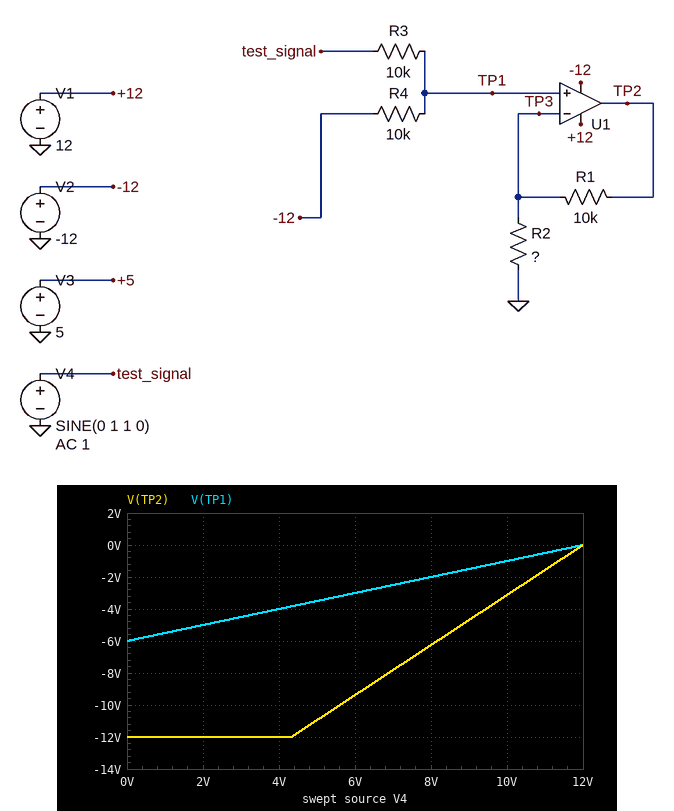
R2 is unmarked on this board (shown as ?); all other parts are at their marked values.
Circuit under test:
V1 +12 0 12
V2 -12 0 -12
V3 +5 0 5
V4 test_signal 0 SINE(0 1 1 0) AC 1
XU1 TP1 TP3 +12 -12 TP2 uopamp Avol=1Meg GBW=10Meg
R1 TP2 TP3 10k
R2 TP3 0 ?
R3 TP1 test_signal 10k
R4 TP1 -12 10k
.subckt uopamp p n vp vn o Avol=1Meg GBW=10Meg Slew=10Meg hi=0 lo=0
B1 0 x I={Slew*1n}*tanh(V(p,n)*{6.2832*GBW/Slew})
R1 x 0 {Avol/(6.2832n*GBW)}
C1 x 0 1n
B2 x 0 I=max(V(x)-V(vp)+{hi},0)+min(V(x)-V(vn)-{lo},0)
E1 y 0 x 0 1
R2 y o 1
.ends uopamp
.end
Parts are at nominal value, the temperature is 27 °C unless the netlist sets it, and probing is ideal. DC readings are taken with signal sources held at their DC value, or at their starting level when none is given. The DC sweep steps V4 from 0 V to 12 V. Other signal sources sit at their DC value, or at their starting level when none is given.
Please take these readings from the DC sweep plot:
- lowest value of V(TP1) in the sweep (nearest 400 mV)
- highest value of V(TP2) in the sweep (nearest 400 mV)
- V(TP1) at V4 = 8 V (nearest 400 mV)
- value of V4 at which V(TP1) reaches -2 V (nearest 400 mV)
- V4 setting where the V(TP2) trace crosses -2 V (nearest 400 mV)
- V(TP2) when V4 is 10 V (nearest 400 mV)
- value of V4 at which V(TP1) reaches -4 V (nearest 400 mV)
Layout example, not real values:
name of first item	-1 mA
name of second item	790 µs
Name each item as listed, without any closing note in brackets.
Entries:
lowest value of V(TP1) in the sweep	-6.0 V
highest value of V(TP2) in the sweep	0 V
V(TP1) at V4 = 8 V	-2.0 V
value of V4 at which V(TP1) reaches -2 V	8.0 V
V4 setting where the V(TP2) trace crosses -2 V	10.8 V
V(TP2) when V4 is 10 V	-3.2 V
value of V4 at which V(TP1) reaches -4 V	4.0 V
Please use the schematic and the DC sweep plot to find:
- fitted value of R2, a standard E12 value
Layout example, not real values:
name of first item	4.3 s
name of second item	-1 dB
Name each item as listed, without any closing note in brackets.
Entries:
fitted value of R2, a standard E12 value	4.7 kΩ
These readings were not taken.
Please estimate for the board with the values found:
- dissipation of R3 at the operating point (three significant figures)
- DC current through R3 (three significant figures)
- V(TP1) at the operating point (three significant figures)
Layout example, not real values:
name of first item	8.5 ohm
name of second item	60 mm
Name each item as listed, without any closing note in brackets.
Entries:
dissipation of R3 at the operating point	3.60 mW
DC current through R3	600 µA
V(TP1) at the operating point	-6.00 V
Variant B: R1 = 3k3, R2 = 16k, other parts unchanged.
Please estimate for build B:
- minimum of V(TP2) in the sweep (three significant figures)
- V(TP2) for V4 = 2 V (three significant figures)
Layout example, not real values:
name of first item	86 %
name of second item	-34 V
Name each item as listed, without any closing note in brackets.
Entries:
minimum of V(TP2) in the sweep	-7.24 V
V(TP2) for V4 = 2 V	-6.03 V
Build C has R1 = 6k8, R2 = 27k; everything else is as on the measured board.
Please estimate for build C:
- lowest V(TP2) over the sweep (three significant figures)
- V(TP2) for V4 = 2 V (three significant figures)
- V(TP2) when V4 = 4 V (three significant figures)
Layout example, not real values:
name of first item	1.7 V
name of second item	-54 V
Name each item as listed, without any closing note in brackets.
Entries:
lowest V(TP2) over the sweep	-7.51 V
V(TP2) for V4 = 2 V	-6.26 V
V(TP2) when V4 = 4 V	-5.01 V
